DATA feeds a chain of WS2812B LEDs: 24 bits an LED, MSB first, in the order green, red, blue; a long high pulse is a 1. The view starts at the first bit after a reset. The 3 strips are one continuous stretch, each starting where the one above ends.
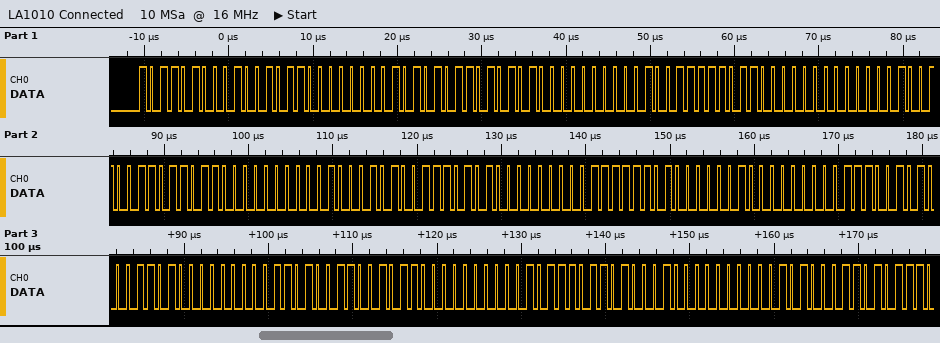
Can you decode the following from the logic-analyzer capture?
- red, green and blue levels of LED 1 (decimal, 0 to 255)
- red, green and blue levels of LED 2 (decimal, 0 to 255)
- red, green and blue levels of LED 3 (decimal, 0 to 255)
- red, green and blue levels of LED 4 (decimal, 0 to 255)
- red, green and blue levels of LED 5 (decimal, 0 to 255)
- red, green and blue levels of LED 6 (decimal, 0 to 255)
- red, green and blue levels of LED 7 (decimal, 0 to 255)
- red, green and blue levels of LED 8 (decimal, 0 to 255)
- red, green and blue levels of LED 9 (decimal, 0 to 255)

75, 180, 0
84, 171, 0
96, 159, 0
108, 147, 0
117, 138, 0
129, 126, 0
141, 114, 0
150, 105, 0
162, 93, 0
